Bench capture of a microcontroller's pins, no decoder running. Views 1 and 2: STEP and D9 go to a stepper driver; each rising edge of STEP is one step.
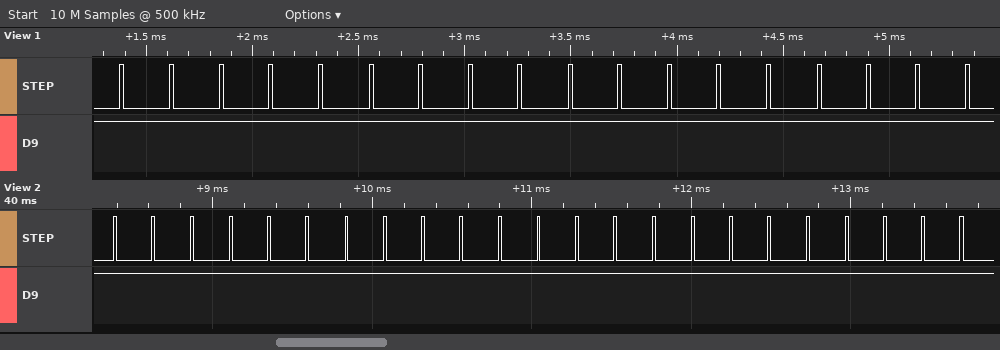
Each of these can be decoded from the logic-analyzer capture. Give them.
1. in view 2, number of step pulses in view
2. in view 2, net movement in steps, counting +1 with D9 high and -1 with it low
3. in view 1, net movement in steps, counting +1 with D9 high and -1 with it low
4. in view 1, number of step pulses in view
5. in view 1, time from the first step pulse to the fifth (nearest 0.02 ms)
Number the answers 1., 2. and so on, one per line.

1. 23
2. +23
3. +18
4. 18
5. 0.94 ms
